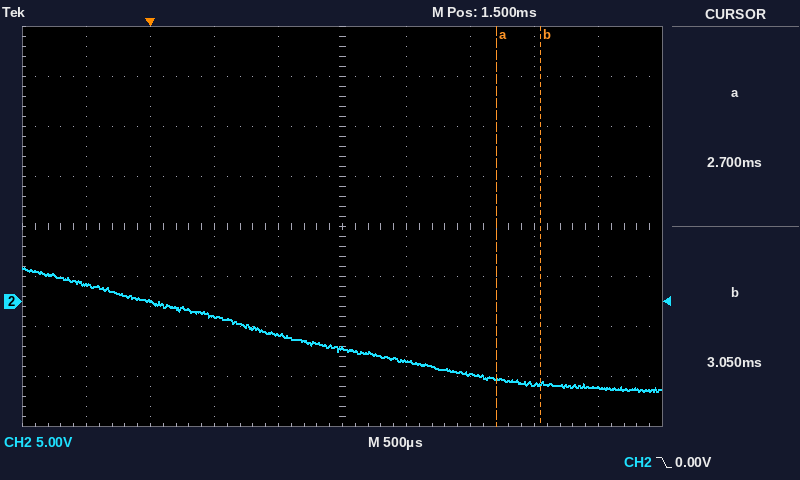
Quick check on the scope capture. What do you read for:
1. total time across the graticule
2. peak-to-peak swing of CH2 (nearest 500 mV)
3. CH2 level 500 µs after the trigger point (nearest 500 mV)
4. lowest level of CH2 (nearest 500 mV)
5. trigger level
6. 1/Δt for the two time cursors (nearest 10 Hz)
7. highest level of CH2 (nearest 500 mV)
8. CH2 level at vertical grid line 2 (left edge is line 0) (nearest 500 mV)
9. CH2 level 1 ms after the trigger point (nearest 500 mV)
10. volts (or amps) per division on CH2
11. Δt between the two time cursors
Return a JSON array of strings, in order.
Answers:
["5 ms", "12.5 V", "-1.5 V", "-9.0 V", "0.00 V", "2.86 kHz", "3.5 V", "0.0 V", "-3.5 V", "5 V", "350 µs"]
